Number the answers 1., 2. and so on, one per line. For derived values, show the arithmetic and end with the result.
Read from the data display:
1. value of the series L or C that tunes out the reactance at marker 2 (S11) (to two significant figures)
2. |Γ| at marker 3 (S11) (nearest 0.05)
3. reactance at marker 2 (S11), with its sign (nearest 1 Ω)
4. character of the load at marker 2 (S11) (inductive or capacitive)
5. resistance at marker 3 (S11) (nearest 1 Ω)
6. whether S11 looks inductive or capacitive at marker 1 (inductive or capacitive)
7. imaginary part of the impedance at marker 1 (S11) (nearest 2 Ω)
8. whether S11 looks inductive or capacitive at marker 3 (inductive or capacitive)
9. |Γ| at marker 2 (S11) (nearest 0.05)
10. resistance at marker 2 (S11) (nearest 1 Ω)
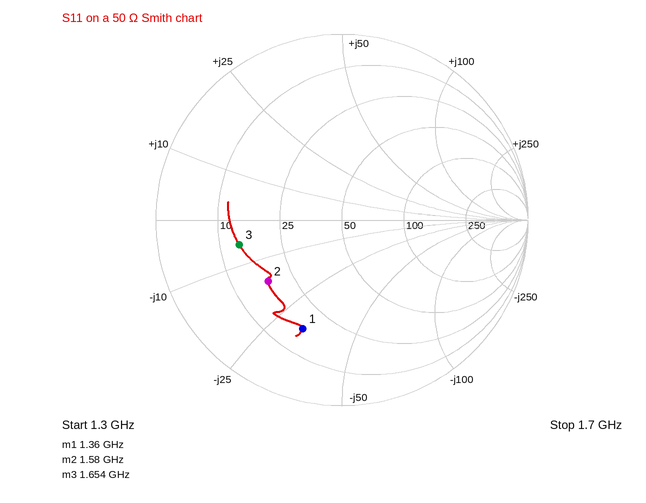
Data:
1. L = 16 Ω/(2π × 1.58 GHz) ≈ 1.6 nH
2. 0.55
3. -16 Ω
4. capacitive
5. 14 Ω
6. capacitive
7. -32 Ω
8. capacitive
9. 0.50
10. 18 Ω
